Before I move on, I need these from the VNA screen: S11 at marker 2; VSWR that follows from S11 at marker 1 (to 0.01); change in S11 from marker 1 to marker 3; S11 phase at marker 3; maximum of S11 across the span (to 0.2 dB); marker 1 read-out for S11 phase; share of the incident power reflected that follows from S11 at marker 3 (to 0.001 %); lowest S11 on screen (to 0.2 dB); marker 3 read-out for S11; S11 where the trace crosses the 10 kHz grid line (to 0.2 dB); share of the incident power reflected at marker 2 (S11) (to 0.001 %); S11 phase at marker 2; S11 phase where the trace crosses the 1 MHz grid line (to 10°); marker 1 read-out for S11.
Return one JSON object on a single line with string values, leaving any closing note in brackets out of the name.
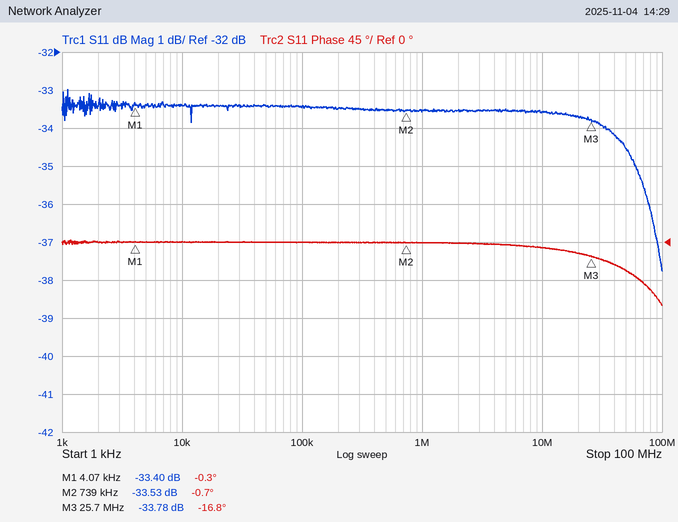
{"S11 at marker 2": "-33.53 dB", "VSWR that follows from S11 at marker 1": "1.04", "change in S11 from marker 1 to marker 3": "-0.38 dB", "S11 phase at marker 3": "-16.8°", "maximum of S11 across the span": "-33.0 dB", "marker 1 read-out for S11 phase": "-0.3°", "share of the incident power reflected that follows from S11 at marker 3": "0.042 %", "lowest S11 on screen": "-37.8 dB", "marker 3 read-out for S11": "-33.78 dB", "S11 where the trace crosses the 10 kHz grid line": "-33.4 dB", "share of the incident power reflected at marker 2 (S11)": "0.044 %", "S11 phase at marker 2": "-0.7°", "S11 phase where the trace crosses the 1 MHz grid line": "0°", "marker 1 read-out for S11": "-33.40 dB"}
